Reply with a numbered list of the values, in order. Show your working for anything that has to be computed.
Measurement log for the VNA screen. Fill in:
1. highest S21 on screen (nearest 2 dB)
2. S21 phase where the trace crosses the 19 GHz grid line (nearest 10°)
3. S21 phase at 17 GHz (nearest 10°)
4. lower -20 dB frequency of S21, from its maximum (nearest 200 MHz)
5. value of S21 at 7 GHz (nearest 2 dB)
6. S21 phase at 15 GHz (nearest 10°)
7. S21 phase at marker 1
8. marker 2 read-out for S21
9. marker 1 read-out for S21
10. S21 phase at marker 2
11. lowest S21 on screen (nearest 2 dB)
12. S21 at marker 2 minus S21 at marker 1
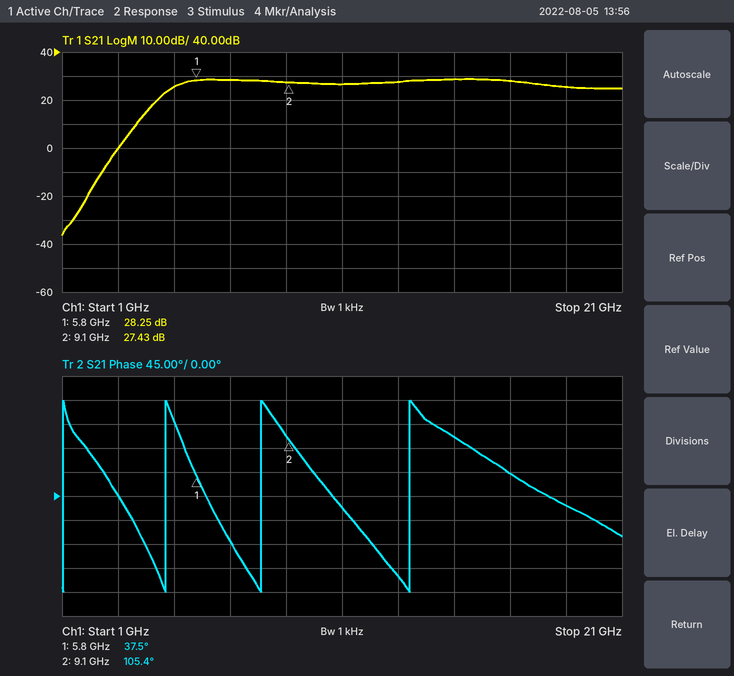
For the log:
1. 28 dB
2. -20°
3. 40°
4. 3.6 GHz
5. 28 dB
6. 110°
7. 37.5°
8. 27.43 dB
9. 28.25 dB
10. 105.4°
11. -36 dB
12. 27.43 − (28.25) = -0.82 dB
